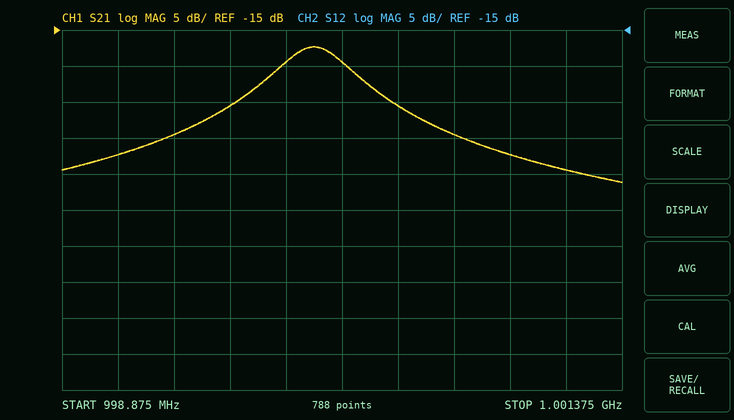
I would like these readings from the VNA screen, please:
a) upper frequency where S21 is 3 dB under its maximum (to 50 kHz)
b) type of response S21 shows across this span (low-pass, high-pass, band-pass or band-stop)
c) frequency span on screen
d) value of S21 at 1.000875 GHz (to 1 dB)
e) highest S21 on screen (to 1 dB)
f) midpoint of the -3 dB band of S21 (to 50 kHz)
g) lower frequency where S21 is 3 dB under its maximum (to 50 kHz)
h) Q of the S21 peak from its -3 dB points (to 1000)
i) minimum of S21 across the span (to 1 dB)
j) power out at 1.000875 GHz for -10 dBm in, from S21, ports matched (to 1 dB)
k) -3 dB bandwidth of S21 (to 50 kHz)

1.00015 GHz
band-pass
2.5 MHz
-32 dB
-17 dB
1.00000 GHz
999.85 MHz
3000
-36 dB
-42 dBm
300 kHz
